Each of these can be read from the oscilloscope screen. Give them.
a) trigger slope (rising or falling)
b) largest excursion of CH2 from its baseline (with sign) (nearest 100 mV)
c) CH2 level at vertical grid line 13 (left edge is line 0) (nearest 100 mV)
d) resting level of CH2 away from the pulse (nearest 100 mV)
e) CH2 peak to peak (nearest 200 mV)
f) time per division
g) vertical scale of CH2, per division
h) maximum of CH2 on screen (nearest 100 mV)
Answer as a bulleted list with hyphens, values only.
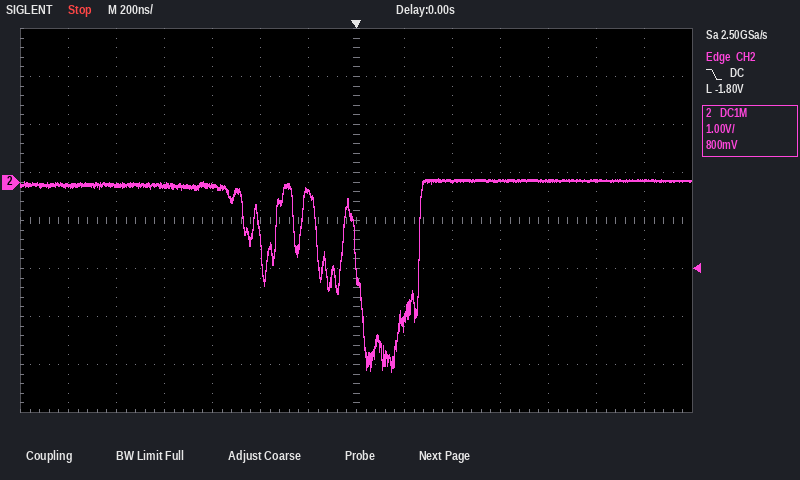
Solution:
- falling
- -4.0 V
- 0.0 V
- 0.0 V
- 4.0 V
- 200 ns
- 1 V
- 100 mV
